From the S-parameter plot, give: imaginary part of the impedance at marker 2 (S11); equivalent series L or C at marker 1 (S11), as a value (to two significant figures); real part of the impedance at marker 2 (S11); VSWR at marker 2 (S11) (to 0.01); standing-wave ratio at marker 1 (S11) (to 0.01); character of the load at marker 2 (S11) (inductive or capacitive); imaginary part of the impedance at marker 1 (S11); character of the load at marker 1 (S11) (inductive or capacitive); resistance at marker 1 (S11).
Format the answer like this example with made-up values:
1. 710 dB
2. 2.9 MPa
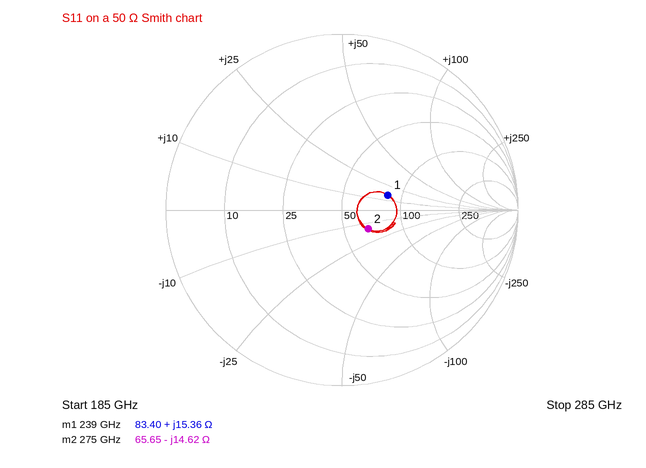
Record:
1. -14.62 Ω
2. 10 pH
3. 65.65 Ω
4. 1.45
5. 1.75
6. capacitive
7. +15.36 Ω
8. inductive
9. 83.40 Ω
